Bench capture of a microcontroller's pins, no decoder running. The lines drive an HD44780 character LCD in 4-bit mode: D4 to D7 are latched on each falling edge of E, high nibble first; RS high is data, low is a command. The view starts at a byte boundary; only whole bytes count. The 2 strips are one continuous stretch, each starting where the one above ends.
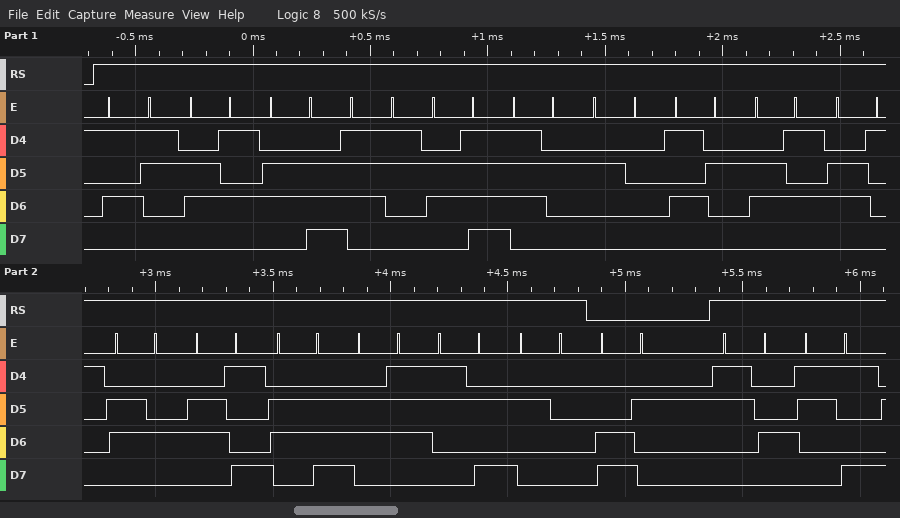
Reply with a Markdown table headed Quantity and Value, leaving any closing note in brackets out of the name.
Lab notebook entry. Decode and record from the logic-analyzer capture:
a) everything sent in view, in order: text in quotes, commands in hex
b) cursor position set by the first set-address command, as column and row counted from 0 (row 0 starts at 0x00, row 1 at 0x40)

| Quantity | Value |
|---|---|
| everything sent in view, in order: text in quotes, commands in hex | "Sensor Reading: " 0xC2 "49" |
| cursor position set by the first set-address command, as column and row counted from 0 | column 2, row 1 |
